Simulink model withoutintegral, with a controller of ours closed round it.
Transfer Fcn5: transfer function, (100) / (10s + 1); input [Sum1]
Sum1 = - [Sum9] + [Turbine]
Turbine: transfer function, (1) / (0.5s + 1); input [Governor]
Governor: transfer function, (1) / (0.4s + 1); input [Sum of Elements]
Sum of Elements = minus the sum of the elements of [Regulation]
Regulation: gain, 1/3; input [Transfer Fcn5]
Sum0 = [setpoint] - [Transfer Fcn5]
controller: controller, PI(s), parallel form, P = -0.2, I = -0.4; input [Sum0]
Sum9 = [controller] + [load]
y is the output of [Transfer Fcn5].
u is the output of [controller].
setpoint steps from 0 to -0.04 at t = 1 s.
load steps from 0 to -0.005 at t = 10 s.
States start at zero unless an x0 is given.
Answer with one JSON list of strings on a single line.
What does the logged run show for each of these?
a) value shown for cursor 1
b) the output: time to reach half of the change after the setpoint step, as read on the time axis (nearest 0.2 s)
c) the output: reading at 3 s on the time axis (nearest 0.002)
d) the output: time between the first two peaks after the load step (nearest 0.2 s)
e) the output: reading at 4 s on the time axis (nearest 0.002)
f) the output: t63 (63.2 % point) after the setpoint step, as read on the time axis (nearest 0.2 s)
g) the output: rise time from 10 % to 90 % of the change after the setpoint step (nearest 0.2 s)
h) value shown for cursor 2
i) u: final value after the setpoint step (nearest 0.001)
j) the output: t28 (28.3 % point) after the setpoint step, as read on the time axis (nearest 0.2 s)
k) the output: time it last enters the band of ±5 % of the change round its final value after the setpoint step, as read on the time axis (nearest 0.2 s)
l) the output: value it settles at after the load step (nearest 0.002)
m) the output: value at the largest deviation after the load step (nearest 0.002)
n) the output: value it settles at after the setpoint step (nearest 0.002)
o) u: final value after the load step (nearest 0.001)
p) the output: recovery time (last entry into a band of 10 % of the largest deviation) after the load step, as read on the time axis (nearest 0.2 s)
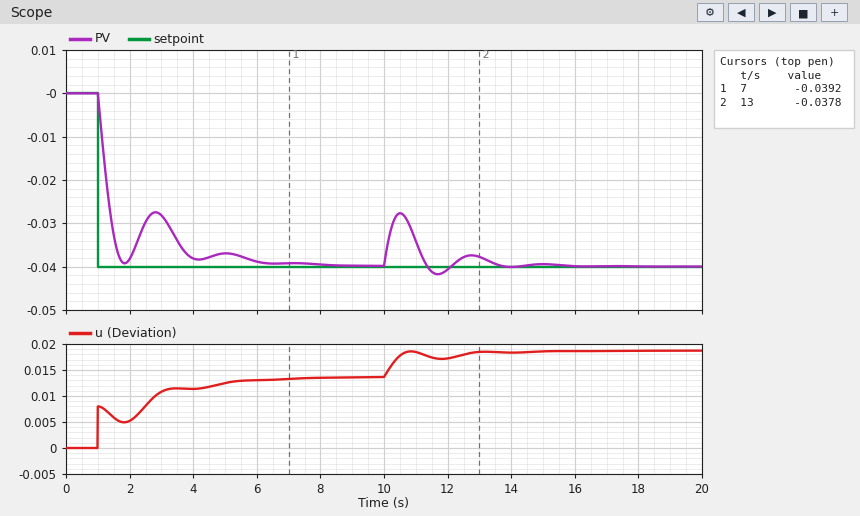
["-0.0392", "1.2 s", "-0.028", "2.2 s", "-0.038", "1.4 s", "0.6 s", "-0.0378", "0.014", "1.2 s", "5.6 s", "-0.040", "-0.028", "-0.040", "0.019", "13.4 s"]
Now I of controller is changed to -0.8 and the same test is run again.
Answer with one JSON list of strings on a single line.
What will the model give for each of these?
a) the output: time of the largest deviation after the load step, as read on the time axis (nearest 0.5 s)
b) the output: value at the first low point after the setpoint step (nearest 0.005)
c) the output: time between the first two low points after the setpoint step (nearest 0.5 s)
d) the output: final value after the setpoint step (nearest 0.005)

["10.5 s", "-0.045", "2.0 s", "-0.040"]
